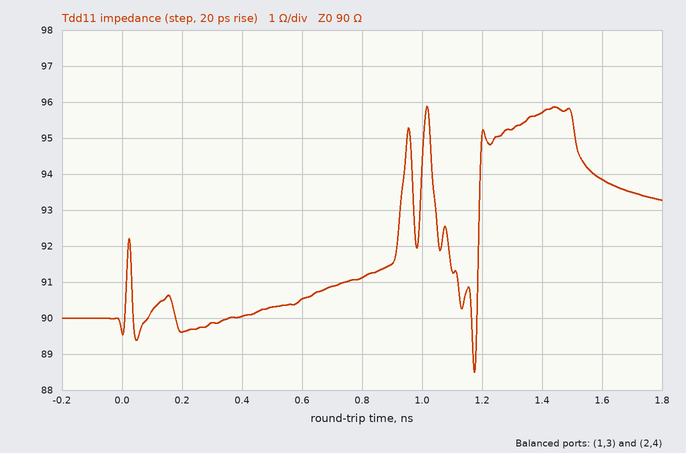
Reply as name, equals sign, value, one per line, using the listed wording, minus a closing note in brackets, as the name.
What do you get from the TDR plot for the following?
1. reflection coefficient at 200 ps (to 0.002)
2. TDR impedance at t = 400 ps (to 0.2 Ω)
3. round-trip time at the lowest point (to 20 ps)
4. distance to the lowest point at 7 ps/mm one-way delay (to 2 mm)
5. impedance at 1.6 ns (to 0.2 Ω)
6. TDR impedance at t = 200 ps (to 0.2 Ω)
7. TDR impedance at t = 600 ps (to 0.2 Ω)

reflection coefficient at 200 ps = -0.002
TDR impedance at t = 400 ps = 90.0 Ω
round-trip time at the lowest point = 1.18 ns
distance to the lowest point at 7 ps/mm one-way delay = 84 mm
impedance at 1.6 ns = 93.8 Ω
TDR impedance at t = 200 ps = 89.6 Ω
TDR impedance at t = 600 ps = 90.6 Ω
